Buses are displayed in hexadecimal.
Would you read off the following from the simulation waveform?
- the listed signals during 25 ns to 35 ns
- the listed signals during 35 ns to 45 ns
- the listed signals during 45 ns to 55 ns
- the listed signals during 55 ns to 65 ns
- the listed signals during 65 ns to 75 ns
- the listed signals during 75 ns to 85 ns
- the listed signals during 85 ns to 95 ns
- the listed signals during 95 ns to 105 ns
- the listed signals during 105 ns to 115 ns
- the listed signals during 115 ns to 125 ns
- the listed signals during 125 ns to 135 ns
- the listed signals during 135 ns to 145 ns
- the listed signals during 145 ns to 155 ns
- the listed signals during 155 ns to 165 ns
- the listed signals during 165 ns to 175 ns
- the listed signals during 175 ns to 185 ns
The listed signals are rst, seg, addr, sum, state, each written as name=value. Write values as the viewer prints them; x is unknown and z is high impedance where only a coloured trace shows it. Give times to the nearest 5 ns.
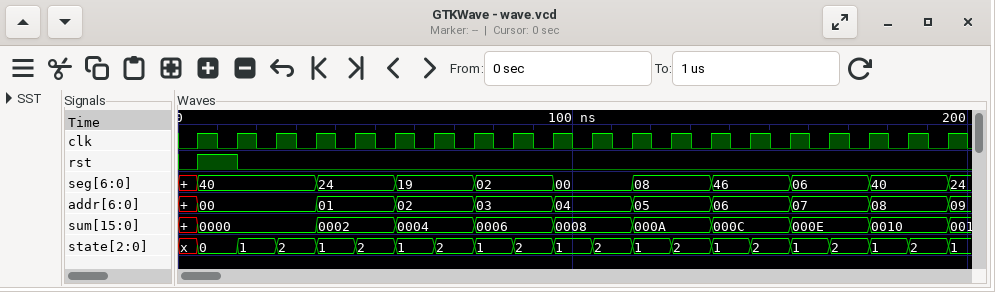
rst=0, seg=40, addr=00, sum=0000, state=2
rst=0, seg=24, addr=01, sum=0002, state=1
rst=0, seg=24, addr=01, sum=0002, state=2
rst=0, seg=19, addr=02, sum=0004, state=1
rst=0, seg=19, addr=02, sum=0004, state=2
rst=0, seg=02, addr=03, sum=0006, state=1
rst=0, seg=02, addr=03, sum=0006, state=2
rst=0, seg=00, addr=04, sum=0008, state=1
rst=0, seg=00, addr=04, sum=0008, state=2
rst=0, seg=08, addr=05, sum=000A, state=1
rst=0, seg=08, addr=05, sum=000A, state=2
rst=0, seg=46, addr=06, sum=000C, state=1
rst=0, seg=46, addr=06, sum=000C, state=2
rst=0, seg=06, addr=07, sum=000E, state=1
rst=0, seg=06, addr=07, sum=000E, state=2
rst=0, seg=40, addr=08, sum=0010, state=1
